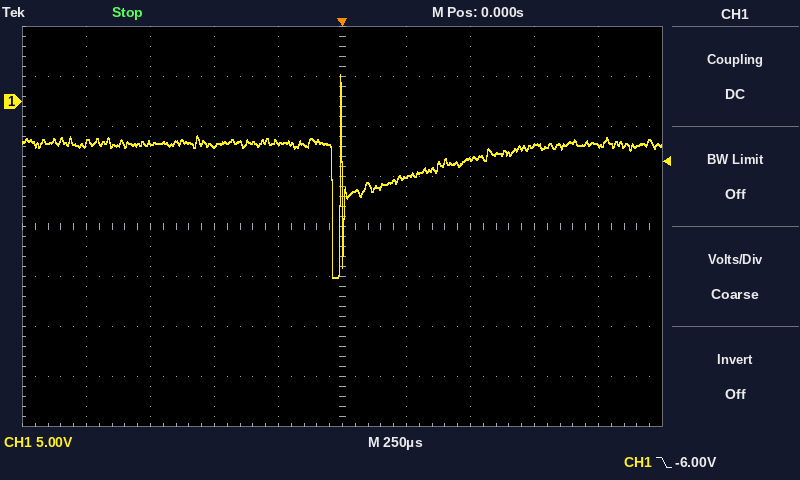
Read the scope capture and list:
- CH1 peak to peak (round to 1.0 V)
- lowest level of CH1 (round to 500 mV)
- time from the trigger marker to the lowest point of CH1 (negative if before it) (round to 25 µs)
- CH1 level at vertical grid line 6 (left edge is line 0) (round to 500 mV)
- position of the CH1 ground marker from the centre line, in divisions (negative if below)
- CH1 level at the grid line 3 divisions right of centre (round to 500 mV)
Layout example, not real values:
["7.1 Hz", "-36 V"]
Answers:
["20.0 V", "-17.5 V", "-25 µs", "-7.5 V", "+2.5 div", "-4.5 V"]
